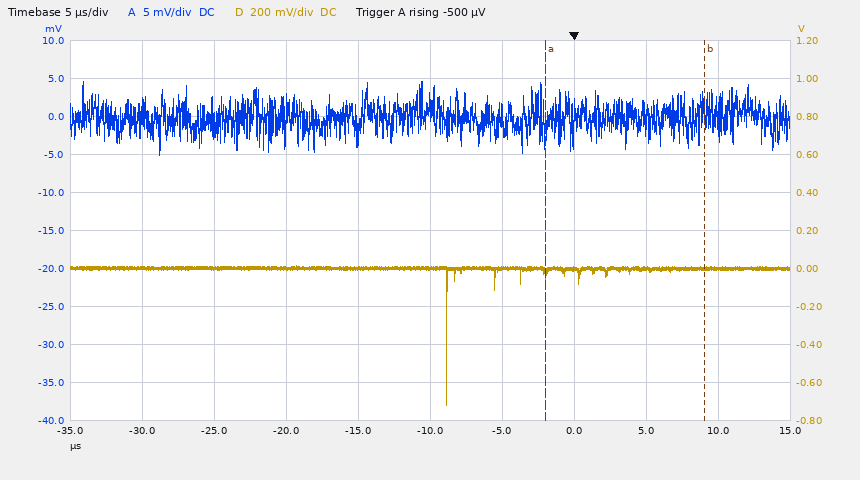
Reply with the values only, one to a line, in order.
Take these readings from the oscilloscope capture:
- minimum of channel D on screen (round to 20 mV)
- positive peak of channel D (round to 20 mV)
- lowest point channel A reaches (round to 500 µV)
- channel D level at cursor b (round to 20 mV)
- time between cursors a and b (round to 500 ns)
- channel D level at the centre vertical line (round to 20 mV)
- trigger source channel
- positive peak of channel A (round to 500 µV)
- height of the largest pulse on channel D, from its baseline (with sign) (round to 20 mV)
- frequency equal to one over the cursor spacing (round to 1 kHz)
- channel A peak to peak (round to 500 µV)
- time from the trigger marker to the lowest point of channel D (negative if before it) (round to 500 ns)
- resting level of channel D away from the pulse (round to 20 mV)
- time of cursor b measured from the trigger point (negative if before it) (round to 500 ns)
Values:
-720 mV
20 mV
-5.0 mV
0 mV
11.0 µs
0 mV
channel A
4.5 mV
-720 mV
91 kHz
9.5 mV
-9.0 µs
0 mV
+9.0 µs
